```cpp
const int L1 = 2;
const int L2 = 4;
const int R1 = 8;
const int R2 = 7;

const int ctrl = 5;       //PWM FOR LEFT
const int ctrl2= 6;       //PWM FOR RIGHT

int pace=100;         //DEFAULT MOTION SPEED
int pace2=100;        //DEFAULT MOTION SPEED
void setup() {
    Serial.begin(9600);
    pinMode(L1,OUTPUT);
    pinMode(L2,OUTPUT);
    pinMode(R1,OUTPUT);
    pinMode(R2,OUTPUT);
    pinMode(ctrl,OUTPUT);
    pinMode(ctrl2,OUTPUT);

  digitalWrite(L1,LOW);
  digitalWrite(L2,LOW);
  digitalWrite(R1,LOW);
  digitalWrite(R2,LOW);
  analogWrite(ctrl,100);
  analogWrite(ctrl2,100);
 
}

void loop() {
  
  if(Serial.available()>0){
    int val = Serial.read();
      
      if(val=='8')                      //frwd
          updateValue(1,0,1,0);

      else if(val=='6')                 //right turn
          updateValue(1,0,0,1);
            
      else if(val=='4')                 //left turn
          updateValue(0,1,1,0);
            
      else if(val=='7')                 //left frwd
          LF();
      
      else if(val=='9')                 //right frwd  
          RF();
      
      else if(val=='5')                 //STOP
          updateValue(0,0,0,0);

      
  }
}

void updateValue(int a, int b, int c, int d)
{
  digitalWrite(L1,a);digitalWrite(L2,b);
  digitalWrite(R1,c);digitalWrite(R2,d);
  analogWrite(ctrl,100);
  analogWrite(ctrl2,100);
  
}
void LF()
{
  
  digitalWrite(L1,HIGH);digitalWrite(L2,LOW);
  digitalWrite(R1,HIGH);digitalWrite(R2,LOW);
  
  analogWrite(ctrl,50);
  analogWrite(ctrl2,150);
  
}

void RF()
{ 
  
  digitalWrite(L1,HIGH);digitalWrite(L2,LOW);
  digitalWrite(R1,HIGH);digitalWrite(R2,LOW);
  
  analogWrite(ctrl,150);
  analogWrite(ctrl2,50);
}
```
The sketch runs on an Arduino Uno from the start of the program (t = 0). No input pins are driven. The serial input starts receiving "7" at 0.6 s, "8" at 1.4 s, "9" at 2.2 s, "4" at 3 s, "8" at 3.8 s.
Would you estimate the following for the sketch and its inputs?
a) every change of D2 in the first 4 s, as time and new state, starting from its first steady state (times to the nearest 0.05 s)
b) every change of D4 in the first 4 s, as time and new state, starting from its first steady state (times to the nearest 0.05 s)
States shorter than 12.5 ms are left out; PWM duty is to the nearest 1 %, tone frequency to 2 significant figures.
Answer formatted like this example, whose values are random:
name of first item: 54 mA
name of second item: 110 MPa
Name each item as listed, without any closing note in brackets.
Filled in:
every change of D2 in the first 4 s, as time and new state, starting from its first steady state: 0 s low; 0.6 s high; 3 s low; 3.8 s high
every change of D4 in the first 4 s, as time and new state, starting from its first steady state: 0 s low; 3 s high; 3.8 s low
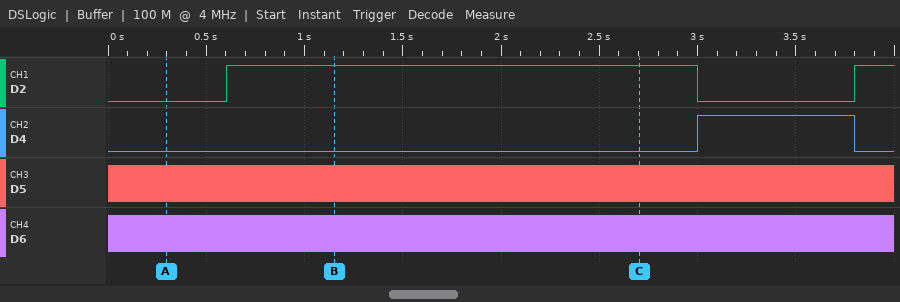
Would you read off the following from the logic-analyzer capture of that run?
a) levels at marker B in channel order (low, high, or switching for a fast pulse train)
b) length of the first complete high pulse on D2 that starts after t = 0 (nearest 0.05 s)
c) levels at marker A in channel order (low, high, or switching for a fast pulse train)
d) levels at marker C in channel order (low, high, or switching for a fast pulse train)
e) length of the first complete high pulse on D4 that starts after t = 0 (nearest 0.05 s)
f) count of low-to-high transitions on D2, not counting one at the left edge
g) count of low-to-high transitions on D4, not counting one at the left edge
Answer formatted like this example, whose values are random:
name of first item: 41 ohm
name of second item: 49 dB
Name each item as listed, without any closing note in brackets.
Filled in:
levels at marker B in channel order: D2 high, D4 low, D5 switching, D6 switching
length of the first complete high pulse on D2 that starts after t = 0: 2.40 s
levels at marker A in channel order: D2 low, D4 low, D5 switching, D6 switching
levels at marker C in channel order: D2 high, D4 low, D5 switching, D6 switching
length of the first complete high pulse on D4 that starts after t = 0: 0.80 s
count of low-to-high transitions on D2, not counting one at the left edge: 2
count of low-to-high transitions on D4, not counting one at the left edge: 1
